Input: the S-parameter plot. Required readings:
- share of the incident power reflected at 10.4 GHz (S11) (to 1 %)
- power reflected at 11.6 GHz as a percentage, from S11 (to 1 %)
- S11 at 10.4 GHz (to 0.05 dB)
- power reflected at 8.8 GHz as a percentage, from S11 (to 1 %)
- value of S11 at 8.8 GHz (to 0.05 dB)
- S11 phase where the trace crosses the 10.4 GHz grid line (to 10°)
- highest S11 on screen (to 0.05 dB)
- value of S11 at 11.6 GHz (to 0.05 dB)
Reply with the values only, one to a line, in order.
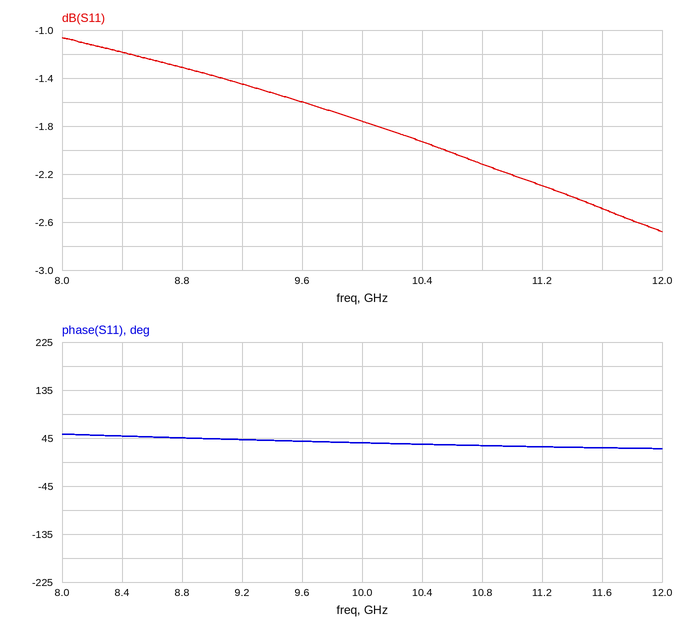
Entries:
64 %
56 %
-1.95 dB
74 %
-1.30 dB
30°
-1.05 dB
-2.50 dB
